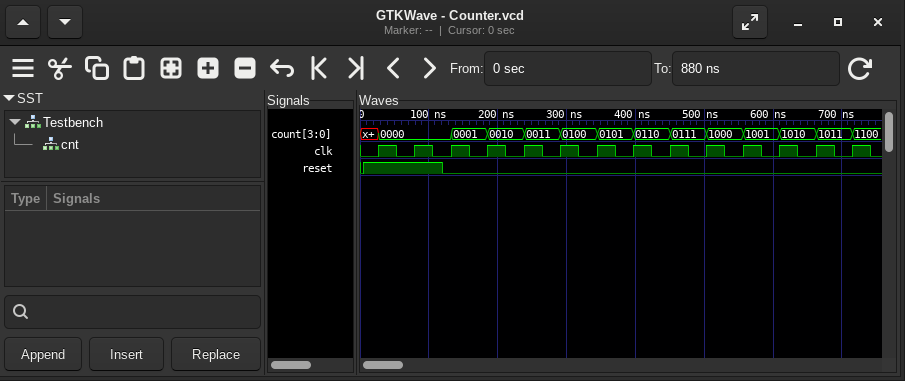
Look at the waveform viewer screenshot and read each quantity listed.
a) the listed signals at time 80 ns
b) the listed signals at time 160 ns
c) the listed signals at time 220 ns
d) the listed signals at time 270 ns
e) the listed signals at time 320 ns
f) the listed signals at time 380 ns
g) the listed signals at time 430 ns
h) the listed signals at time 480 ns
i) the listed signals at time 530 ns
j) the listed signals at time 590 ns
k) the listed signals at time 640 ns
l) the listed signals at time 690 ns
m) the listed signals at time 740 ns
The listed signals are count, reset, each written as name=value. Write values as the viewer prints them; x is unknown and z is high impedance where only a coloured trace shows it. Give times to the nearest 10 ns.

count=0000, reset=1
count=0001, reset=0
count=0010, reset=0
count=0011, reset=0
count=0100, reset=0
count=0101, reset=0
count=0110, reset=0
count=0111, reset=0
count=1000, reset=0
count=1001, reset=0
count=1010, reset=0
count=1011, reset=0
count=1100, reset=0
